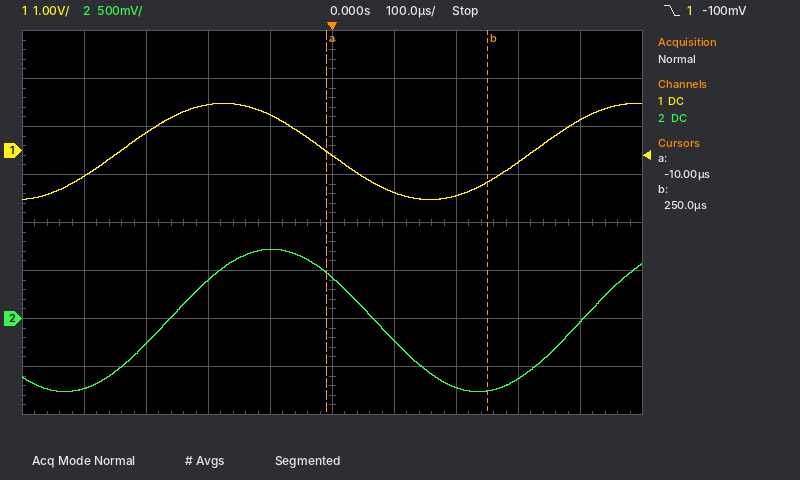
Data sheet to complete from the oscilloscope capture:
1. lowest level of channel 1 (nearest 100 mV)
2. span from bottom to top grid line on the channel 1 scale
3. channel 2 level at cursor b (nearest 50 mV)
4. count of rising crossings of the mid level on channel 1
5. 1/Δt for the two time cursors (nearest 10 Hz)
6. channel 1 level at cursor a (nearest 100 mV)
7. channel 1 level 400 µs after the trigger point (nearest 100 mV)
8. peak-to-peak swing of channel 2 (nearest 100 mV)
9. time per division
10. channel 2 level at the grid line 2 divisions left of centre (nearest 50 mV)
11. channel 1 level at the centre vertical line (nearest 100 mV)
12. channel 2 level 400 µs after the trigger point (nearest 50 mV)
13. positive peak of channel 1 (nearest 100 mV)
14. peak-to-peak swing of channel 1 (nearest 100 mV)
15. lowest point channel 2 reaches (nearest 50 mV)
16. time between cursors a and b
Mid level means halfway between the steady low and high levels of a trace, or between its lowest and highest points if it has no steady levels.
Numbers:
-1.0 V
8 V
-750 mV
2
3.85 kHz
0.0 V
600 mV
1.50 V
100 µs
400 mV
-100 mV
-50 mV
1.0 V
2.0 V
-750 mV
260 µs
